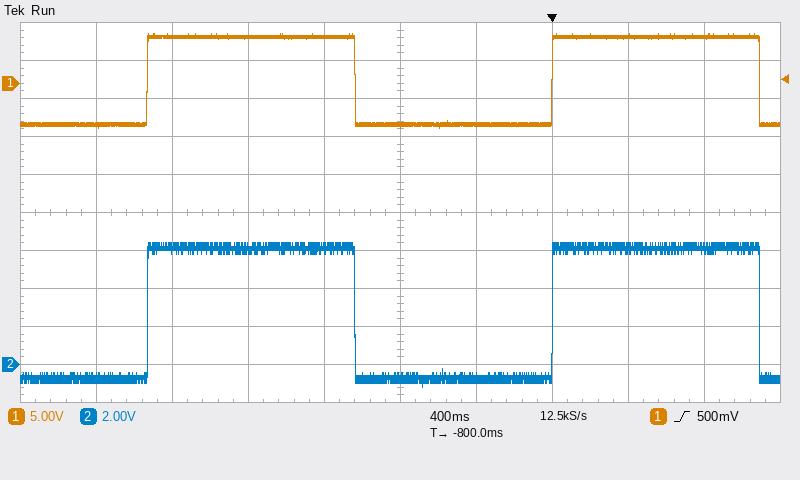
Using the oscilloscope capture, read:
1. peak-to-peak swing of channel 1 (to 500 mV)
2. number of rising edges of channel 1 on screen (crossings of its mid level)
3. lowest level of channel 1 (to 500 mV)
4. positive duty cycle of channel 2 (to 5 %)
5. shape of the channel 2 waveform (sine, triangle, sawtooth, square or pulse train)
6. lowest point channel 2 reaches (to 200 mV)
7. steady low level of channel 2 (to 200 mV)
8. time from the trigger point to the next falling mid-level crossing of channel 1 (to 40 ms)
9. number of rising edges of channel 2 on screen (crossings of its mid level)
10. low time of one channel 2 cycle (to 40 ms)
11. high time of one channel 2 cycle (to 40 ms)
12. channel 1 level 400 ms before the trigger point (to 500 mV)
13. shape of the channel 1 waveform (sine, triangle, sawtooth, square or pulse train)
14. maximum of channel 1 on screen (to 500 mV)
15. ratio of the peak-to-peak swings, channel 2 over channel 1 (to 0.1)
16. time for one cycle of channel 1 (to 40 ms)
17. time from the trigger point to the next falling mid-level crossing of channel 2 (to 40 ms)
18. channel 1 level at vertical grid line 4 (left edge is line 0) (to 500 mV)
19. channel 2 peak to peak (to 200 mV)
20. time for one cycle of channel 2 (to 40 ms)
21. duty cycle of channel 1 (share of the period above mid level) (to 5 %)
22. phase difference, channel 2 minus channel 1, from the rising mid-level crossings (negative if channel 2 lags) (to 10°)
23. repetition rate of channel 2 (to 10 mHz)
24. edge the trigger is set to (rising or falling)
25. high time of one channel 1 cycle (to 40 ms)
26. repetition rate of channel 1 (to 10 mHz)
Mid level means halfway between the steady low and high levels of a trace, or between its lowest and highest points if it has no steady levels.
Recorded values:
12.5 V
2
-6.0 V
50 %
square
-1.2 V
-800 mV
1.08 s
2
1.04 s
1.08 s
-5.5 V
square
6.5 V
0.6
2.12 s
1.08 s
6.0 V
7.6 V
2.12 s
50 %
0°
470 mHz
rising
1.08 s
470 mHz
